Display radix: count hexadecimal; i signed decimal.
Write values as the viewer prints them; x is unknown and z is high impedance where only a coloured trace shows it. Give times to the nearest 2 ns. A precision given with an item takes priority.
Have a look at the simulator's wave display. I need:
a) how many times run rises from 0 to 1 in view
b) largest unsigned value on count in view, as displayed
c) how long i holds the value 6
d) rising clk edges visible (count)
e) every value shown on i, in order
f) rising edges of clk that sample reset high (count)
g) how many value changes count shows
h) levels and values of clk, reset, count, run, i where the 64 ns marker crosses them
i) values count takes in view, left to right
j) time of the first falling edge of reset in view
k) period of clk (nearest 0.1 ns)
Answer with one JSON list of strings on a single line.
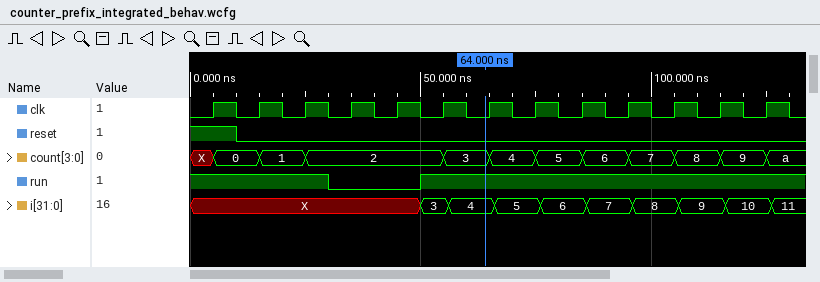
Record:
["1", "a", "10 ns", "13", "X, 3, 4, 5, 6, 7, 8, 9, 10, 11", "1", "11", "clk=0, reset=0, count=3, run=1, i=4", "X, 0, 1, 2, 3, 4, 5, 6, 7, 8, 9, a", "10 ns", "10 ns"]
